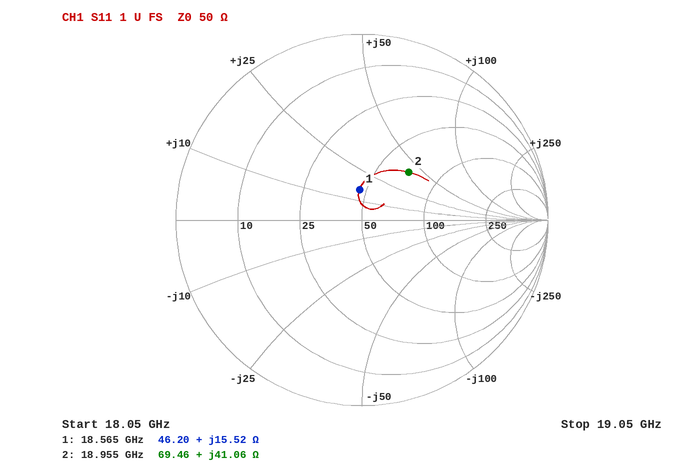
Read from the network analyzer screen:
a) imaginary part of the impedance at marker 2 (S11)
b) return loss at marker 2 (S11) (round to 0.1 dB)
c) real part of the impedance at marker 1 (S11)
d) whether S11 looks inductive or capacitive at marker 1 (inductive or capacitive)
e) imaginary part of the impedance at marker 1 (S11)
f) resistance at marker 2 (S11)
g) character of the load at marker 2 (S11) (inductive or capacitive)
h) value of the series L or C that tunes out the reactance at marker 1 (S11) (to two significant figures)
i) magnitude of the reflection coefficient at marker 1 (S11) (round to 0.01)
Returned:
+41.06 Ω
8.9 dB
46.20 Ω
inductive
+15.52 Ω
69.46 Ω
inductive
550 fF
0.16
